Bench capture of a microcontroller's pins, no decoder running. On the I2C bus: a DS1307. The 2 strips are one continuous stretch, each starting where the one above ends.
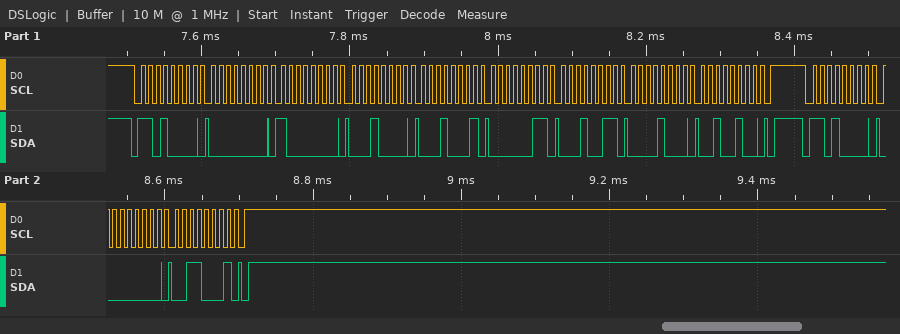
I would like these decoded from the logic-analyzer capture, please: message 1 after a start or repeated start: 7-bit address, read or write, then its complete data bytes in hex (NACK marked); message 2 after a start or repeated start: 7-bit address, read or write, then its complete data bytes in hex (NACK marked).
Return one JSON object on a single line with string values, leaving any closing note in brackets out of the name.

{"message 1 after a start or repeated start: 7-bit address, read or write, then its complete data bytes in hex": "0x68 write: 00 80 10 11 03 13 08 24", "message 2 after a start or repeated start: 7-bit address, read or write, then its complete data bytes in hex": "0x68 write: 00 31"}
